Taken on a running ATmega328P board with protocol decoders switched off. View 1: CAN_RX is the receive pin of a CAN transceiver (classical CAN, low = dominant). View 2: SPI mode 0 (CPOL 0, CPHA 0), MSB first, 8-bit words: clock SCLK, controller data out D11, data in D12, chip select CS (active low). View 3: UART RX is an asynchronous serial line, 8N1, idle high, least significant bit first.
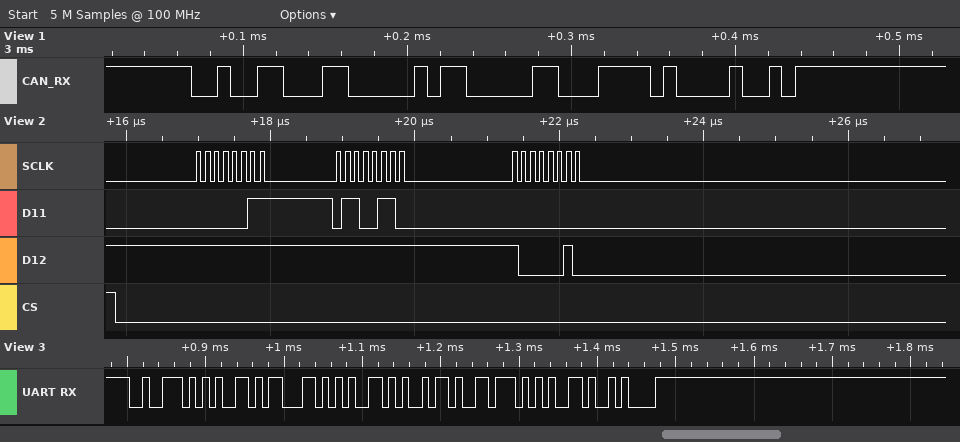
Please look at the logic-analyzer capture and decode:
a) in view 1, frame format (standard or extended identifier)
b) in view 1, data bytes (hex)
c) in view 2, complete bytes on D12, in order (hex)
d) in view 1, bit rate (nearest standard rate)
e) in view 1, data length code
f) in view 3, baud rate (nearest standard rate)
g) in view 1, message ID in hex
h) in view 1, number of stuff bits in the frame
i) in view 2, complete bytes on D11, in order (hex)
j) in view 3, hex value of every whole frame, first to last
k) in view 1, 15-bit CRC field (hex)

standard
82
FF FF 82
125 kbit/s
1
115200 baud
0x263
2
03 66 00
72 65 63 65 69 76 65 0A
0x1E84
